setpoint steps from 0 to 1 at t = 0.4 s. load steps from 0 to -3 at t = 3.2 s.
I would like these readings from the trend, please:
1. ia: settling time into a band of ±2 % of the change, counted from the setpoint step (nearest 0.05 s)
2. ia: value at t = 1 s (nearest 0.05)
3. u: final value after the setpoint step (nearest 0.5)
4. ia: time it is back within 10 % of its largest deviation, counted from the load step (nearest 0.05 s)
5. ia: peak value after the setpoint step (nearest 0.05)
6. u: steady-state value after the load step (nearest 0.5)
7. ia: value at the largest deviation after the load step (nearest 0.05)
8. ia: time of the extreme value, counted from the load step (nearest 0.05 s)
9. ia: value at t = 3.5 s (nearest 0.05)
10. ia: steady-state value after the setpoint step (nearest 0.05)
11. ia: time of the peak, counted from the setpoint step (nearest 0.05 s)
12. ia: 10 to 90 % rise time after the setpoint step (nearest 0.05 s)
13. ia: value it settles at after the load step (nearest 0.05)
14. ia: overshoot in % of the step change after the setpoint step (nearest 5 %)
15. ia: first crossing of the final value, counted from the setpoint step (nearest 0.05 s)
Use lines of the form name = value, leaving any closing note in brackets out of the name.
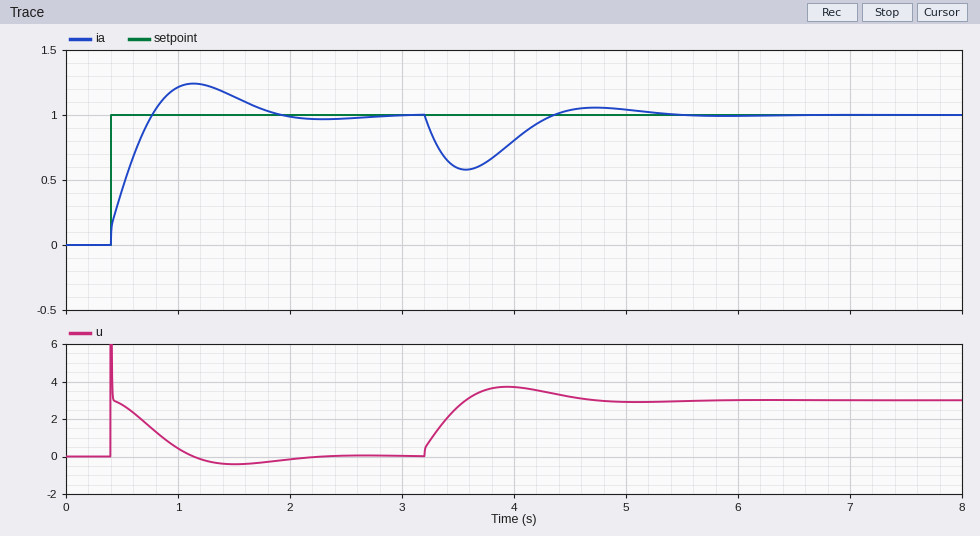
ia: settling time into a band of ±2 % of the change, counted from the setpoint step = 2.25 s
ia: value at t = 1 s = 1.20
u: final value after the setpoint step = 0.0
ia: time it is back within 10 % of its largest deviation, counted from the load step = 1.80 s
ia: peak value after the setpoint step = 1.25
u: steady-state value after the load step = 3.0
ia: value at the largest deviation after the load step = 0.60
ia: time of the extreme value, counted from the load step = 0.35 s
ia: value at t = 3.5 s = 0.60
ia: steady-state value after the setpoint step = 1.00
ia: time of the peak, counted from the setpoint step = 0.75 s
ia: 10 to 90 % rise time after the setpoint step = 0.30 s
ia: value it settles at after the load step = 1.00
ia: overshoot in % of the step change after the setpoint step = 25 %
ia: first crossing of the final value, counted from the setpoint step = 0.35 s
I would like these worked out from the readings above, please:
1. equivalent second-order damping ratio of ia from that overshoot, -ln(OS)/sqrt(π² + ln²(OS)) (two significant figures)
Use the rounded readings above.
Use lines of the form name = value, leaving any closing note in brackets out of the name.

equivalent second-order damping ratio of ia from that overshoot, -ln(OS)/sqrt(π² + ln²(OS)) = 0.40
